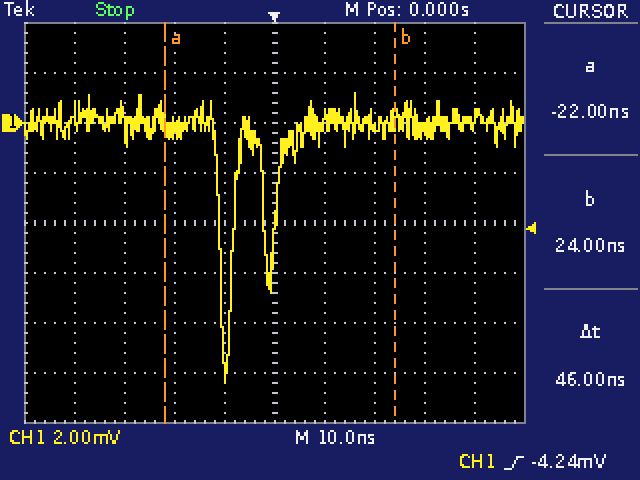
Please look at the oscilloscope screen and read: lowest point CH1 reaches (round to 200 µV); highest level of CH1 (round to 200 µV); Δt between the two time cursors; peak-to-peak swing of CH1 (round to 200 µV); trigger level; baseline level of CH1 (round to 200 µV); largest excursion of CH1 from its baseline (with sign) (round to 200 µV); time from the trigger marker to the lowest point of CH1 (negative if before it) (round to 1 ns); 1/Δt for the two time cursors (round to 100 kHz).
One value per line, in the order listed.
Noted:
-10.4 mV
1.2 mV
46 ns
11.6 mV
-4.24 mV
0.0 mV
-10.4 mV
-10 ns
21.7 MHz
